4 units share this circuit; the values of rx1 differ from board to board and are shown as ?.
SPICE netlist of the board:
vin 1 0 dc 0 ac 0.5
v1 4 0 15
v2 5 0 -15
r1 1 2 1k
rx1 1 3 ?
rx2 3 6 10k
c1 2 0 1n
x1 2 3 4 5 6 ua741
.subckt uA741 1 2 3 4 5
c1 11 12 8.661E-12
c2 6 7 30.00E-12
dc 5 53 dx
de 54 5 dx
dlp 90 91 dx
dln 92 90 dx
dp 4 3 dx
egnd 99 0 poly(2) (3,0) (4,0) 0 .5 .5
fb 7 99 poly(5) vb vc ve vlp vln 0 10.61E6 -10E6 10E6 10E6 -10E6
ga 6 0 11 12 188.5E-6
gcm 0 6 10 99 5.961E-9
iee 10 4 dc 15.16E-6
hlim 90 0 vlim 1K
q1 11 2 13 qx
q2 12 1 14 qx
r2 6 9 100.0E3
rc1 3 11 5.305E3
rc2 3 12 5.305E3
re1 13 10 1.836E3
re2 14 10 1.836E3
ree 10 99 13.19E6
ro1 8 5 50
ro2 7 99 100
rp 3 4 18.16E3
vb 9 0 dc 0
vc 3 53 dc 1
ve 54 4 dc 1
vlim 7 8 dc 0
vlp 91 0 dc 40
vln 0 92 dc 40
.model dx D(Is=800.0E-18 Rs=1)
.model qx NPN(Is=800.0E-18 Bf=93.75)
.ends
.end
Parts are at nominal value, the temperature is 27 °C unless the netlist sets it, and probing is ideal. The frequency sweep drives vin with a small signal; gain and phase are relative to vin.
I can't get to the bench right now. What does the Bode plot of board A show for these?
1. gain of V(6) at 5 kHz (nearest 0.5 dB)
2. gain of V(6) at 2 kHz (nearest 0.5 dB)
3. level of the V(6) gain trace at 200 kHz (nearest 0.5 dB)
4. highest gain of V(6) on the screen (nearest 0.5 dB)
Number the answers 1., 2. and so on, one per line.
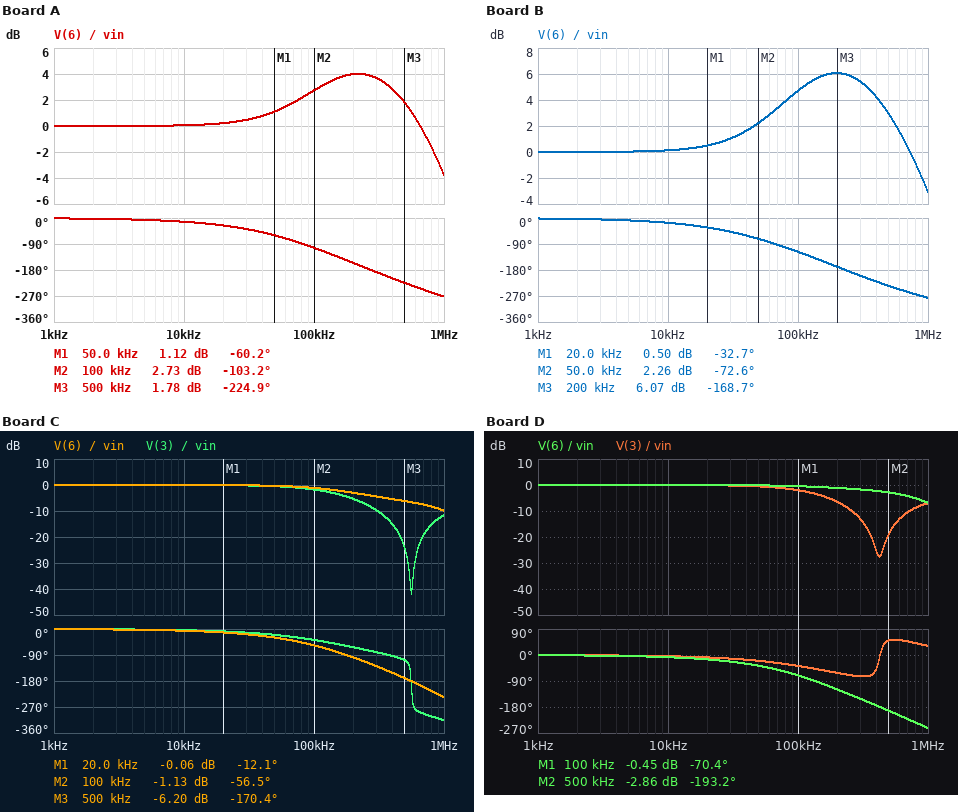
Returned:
1. 0 dB
2. 0 dB
3. 4.0 dB
4. 4.0 dB
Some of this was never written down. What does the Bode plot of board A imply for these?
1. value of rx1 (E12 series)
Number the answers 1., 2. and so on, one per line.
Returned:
1. 4.7 kΩ
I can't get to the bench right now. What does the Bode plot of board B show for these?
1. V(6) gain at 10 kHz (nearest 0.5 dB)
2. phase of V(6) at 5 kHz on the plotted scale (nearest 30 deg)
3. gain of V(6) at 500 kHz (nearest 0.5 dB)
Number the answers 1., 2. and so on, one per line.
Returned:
1. 0 dB
2. 0 deg
3. 3.0 dB
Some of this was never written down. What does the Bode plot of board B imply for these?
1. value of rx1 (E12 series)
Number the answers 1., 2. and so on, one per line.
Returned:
1. 3.3 kΩ
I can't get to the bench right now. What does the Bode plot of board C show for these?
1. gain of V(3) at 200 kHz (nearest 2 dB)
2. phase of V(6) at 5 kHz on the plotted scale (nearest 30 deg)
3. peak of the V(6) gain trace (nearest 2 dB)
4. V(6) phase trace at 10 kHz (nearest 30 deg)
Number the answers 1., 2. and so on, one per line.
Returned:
1. -6 dB
2. 0 deg
3. 0 dB
4. 0 deg
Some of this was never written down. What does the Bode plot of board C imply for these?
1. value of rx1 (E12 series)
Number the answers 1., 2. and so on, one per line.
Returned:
1. 22 kΩ
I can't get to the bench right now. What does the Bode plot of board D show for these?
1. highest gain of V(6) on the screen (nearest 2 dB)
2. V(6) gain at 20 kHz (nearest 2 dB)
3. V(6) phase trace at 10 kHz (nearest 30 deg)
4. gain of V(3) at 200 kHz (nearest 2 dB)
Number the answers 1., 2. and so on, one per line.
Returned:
1. 0 dB
2. 0 dB
3. 0 deg
4. -6 dB
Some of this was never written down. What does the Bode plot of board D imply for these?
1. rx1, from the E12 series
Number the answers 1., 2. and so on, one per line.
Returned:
1. 12 kΩ
